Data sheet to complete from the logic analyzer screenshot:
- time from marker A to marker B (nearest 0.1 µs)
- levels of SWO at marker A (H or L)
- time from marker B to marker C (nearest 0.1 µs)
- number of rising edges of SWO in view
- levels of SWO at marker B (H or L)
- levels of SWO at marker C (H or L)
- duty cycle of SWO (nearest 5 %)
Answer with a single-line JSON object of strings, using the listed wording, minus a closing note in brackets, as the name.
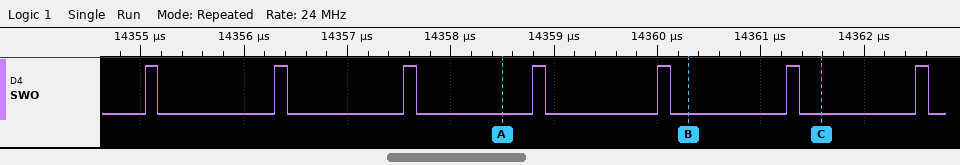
{"time from marker A to marker B": "1.8 µs", "levels of SWO at marker A": "SWO=L", "time from marker B to marker C": "1.3 µs", "number of rising edges of SWO in view": "7", "levels of SWO at marker B": "SWO=L", "levels of SWO at marker C": "SWO=L", "duty cycle of SWO": "10 %"}
